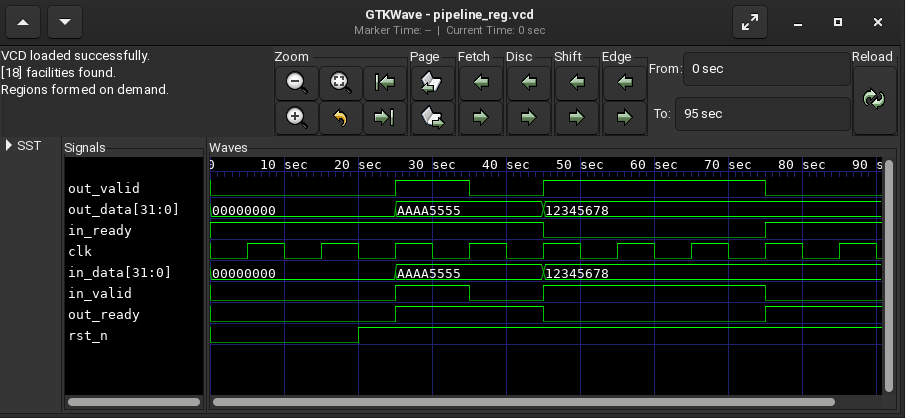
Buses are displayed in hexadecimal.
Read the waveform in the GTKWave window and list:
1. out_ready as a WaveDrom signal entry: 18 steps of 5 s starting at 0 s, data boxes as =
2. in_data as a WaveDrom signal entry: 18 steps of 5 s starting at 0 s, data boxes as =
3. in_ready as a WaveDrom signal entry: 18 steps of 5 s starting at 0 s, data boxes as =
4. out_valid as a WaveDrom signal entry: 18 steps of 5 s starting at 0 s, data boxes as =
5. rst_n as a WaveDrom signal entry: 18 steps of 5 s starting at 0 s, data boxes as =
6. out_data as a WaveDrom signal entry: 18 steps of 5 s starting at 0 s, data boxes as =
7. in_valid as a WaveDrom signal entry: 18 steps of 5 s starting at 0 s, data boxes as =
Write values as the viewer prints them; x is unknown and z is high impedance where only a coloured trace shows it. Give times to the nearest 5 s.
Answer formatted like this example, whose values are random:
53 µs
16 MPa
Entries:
{name: 'out_ready', wave: '0....1...0.....1..'}
{name: 'in_data', wave: '=....=...=........', data: '00000000 AAAA5555 12345678'}
{name: 'in_ready', wave: '1........0.....1..'}
{name: 'out_valid', wave: '0....1.0.1.....0..'}
{name: 'rst_n', wave: '0...1.............'}
{name: 'out_data', wave: '=....=...=........', data: '00000000 AAAA5555 12345678'}
{name: 'in_valid', wave: '0....1.0.1.....0..'}
